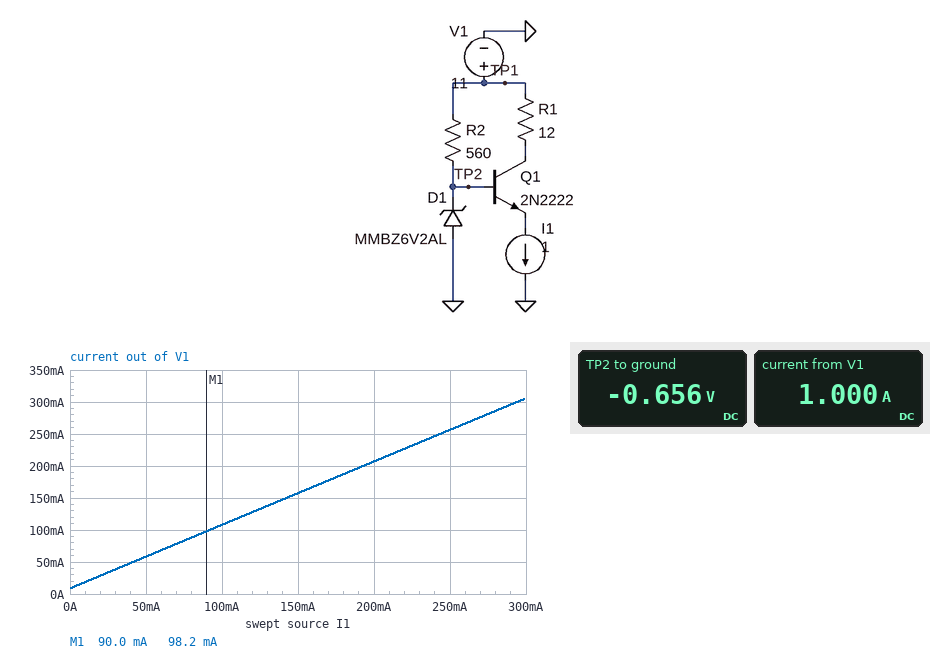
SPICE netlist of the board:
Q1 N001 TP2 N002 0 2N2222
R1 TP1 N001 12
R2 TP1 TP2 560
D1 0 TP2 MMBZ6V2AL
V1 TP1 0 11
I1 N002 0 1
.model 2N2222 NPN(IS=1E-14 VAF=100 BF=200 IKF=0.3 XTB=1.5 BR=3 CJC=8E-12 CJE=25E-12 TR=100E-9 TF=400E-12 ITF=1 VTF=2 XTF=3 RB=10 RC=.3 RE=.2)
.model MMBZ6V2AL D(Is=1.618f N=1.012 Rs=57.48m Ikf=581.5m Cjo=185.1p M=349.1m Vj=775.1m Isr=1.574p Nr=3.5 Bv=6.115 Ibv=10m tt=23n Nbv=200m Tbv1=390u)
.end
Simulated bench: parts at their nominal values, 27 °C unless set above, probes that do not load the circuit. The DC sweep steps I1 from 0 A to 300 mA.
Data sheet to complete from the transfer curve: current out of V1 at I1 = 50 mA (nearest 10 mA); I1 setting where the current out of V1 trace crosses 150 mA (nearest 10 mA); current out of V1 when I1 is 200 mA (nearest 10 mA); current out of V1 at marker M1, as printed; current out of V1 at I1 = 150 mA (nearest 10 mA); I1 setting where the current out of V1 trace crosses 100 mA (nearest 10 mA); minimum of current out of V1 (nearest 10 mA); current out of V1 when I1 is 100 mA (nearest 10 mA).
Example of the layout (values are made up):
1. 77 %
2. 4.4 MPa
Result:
1. 60 mA
2. 140 mA
3. 210 mA
4. 98.2 mA
5. 160 mA
6. 90 mA
7. 10 mA
8. 110 mA
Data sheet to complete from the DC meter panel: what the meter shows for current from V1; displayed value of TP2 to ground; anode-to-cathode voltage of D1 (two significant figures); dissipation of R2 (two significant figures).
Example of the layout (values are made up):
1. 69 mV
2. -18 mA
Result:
1. 1.000 A
2. -0.656 V
3. 660 mV
4. 240 mW
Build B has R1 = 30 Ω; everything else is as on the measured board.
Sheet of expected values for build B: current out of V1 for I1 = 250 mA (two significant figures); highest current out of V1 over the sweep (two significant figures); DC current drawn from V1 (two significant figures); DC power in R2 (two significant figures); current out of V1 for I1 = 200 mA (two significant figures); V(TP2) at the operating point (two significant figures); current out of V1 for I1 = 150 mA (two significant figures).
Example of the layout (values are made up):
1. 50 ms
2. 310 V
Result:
1. 250 mA
2. 300 mA
3. 590 mA
4. 250 mW
5. 200 mA
6. -910 mV
7. 160 mA
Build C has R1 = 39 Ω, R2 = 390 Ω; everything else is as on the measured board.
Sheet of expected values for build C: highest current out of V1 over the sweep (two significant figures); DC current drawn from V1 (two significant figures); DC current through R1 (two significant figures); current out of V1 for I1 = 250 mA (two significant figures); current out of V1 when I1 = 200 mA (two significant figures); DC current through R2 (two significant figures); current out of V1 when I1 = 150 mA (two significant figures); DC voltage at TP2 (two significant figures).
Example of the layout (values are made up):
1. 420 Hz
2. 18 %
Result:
1. 300 mA
2. 490 mA
3. 460 mA
4. 250 mA
5. 200 mA
6. 31 mA
7. 160 mA
8. -930 mV
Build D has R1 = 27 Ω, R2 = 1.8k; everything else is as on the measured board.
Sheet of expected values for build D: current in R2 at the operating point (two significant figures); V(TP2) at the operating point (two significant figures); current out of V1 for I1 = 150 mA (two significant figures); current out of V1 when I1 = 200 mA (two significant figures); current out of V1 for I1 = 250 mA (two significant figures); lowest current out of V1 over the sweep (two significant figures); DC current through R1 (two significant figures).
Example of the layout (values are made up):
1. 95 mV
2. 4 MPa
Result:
1. 6.6 mA
2. -910 mV
3. 150 mA
4. 200 mA
5. 250 mA
6. 2.7 mA
7. 610 mA
